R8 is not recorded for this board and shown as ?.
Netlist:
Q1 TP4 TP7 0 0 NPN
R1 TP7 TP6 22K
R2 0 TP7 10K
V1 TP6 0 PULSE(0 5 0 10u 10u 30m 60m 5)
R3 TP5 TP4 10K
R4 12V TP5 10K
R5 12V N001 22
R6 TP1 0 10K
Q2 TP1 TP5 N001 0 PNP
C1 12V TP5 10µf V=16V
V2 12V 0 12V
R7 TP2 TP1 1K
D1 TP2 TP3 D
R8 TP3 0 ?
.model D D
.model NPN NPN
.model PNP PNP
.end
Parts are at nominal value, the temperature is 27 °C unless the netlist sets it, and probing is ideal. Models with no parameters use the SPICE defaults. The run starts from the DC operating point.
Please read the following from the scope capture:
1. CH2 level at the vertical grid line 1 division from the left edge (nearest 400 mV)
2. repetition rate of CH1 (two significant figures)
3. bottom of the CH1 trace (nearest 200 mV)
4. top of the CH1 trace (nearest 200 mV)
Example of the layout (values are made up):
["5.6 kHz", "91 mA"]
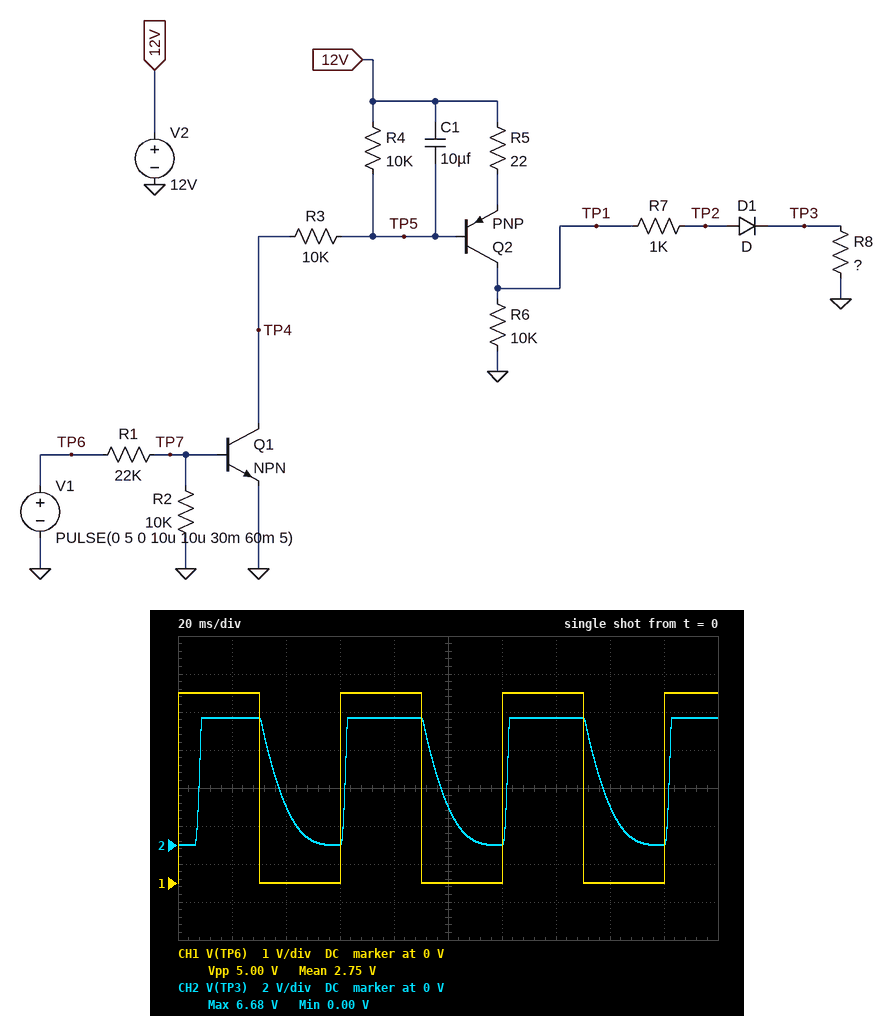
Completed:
["6.8 V", "17 Hz", "0 V", "5.0 V"]
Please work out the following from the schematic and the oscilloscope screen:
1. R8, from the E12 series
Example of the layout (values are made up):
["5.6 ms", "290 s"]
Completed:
["1.5 kΩ"]
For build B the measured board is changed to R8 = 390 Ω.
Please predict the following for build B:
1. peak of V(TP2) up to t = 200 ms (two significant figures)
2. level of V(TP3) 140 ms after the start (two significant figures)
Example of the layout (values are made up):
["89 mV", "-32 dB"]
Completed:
["3.8 V", "3.1 V"]
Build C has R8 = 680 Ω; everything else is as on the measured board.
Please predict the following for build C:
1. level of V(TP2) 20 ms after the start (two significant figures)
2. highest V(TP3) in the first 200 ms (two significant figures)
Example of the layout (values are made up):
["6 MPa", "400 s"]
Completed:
["5.2 V", "4.5 V"]
